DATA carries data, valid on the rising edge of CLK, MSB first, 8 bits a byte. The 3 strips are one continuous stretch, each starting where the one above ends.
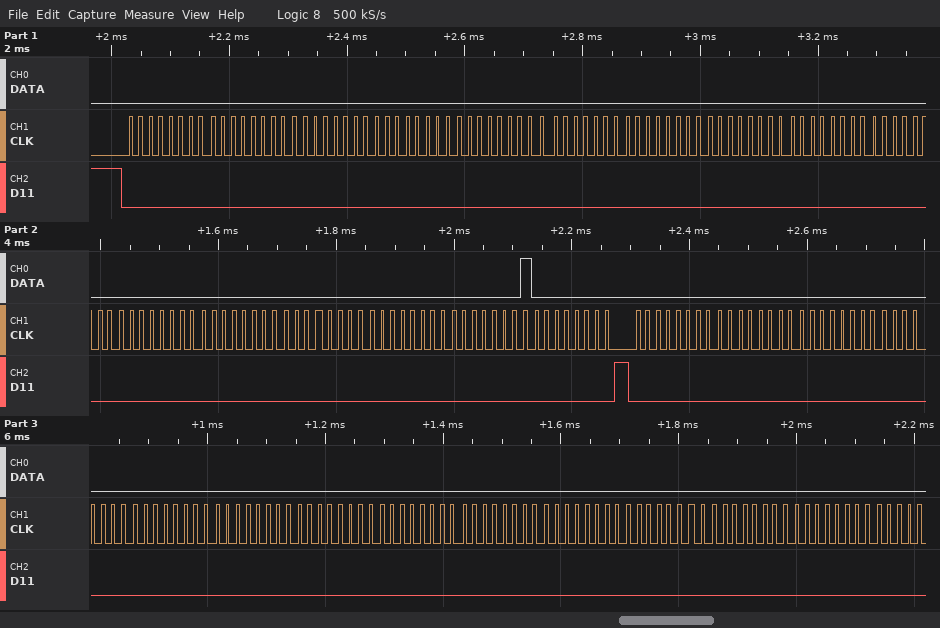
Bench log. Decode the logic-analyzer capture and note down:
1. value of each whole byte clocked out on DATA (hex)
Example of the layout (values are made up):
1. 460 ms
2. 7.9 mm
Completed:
1. 0x00 0x00 0x00 0x00 0x00 0x00 0x00 0x00 0x00 0x00 0x00 0x00 0x00 0x00 0x01 0x00 0x00 0x00 0x00 0x00 0x00 0x00 0x00 0x00 0x00 0x00 0x00 0x00 0x00
